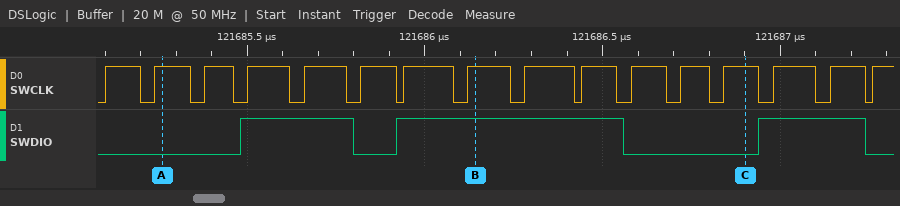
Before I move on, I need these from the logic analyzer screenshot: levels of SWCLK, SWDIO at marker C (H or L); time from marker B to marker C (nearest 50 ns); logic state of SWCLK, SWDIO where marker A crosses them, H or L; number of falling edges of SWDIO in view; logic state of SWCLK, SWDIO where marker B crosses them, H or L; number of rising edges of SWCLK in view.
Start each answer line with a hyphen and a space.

- SWCLK=H, SWDIO=L
- 750 ns
- SWCLK=H, SWDIO=L
- 3
- SWCLK=H, SWDIO=H
- 16
